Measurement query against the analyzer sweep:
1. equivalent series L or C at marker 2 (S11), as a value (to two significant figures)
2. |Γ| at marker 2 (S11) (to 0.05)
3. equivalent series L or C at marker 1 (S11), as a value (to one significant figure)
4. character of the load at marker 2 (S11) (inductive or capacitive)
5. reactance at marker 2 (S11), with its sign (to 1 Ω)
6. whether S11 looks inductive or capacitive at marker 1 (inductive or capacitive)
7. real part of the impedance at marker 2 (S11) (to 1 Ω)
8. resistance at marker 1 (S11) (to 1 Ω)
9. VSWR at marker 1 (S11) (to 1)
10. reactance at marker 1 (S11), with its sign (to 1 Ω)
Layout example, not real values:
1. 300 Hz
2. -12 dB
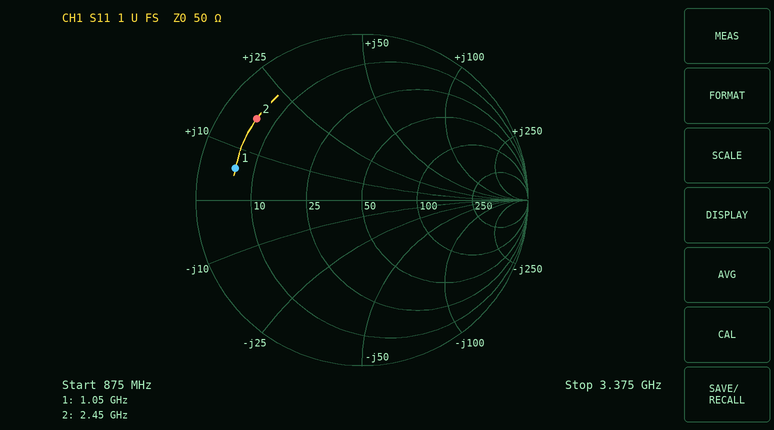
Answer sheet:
1. 1.1 nH
2. 0.80
3. 900 pH
4. inductive
5. +17 Ω
6. inductive
7. 6 Ω
8. 6 Ω
9. 8
10. +6 Ω
